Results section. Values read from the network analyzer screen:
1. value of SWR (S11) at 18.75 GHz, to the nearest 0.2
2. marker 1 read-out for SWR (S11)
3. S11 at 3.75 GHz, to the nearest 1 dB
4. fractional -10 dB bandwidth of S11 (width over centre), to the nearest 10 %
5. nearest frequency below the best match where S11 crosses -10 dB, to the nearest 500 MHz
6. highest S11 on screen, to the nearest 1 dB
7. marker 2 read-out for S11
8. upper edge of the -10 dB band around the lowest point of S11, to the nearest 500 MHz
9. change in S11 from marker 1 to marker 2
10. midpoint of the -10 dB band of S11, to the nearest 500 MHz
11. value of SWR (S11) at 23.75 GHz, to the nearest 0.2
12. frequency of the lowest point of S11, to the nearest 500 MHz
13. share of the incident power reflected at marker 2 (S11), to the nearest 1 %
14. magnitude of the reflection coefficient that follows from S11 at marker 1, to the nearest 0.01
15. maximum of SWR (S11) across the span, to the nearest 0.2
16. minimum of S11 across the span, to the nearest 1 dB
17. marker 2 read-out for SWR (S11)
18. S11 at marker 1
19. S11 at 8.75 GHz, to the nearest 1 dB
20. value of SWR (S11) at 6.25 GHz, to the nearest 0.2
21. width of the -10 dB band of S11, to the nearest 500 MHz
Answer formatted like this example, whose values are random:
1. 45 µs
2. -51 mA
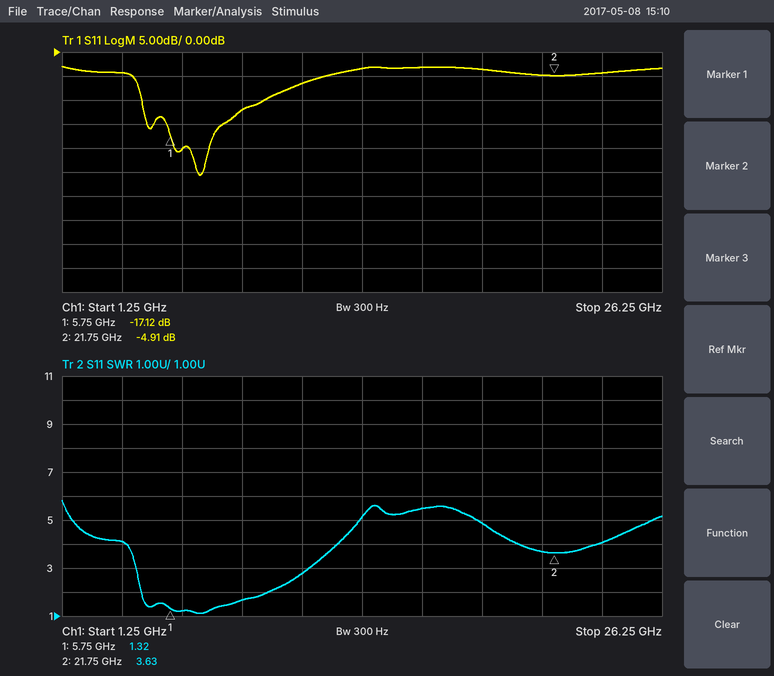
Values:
1. 4.8
2. 1.32
3. -4 dB
4. 70 %
5. 4.5 GHz
6. -3 dB
7. -4.91 dB
8. 9.5 GHz
9. 12.21 dB
10. 7.0 GHz
11. 4.0
12. 7.0 GHz
13. 32 %
14. 0.14
15. 5.8
16. -26 dB
17. 3.63
18. -17.12 dB
19. -12 dB
20. 1.2
21. 5.0 GHz
